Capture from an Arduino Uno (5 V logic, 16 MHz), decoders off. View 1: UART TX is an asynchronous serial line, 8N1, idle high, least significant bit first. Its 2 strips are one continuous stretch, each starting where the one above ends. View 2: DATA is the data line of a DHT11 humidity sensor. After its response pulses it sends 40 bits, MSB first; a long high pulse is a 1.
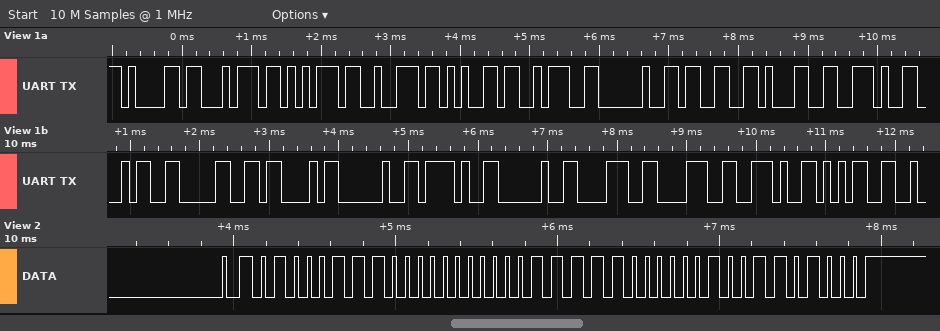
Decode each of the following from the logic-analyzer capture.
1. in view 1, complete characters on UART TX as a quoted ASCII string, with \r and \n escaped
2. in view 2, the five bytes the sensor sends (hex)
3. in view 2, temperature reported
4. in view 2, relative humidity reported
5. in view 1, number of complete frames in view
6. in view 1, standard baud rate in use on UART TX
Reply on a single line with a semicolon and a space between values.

"ature: 31.40C / 88.5"; 47 00 1F 02 68; 31.2 °C; 71 %; 20; 9600 baud
